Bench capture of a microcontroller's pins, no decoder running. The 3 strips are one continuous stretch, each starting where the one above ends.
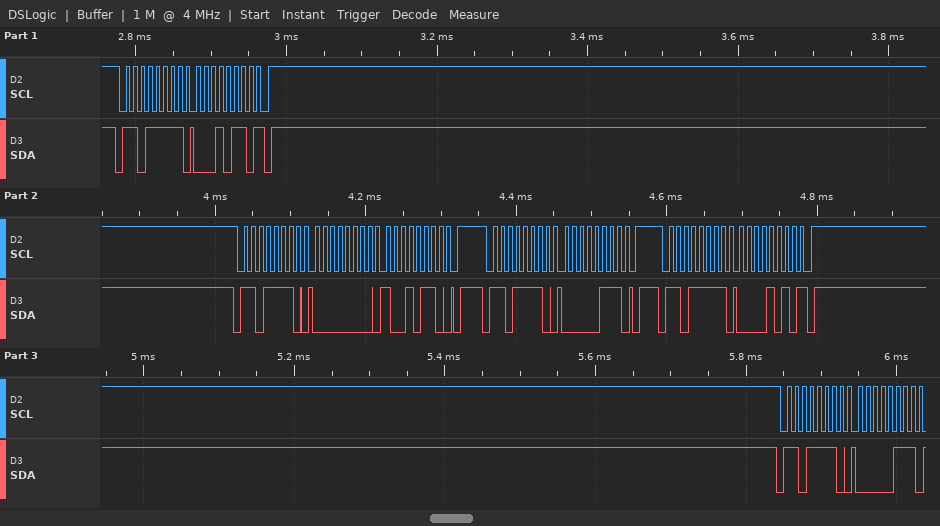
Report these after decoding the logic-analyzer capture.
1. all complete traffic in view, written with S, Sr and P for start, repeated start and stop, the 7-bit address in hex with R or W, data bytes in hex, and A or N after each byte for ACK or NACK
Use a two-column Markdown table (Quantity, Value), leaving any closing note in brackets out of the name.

| Quantity | Value |
|---|---|
| all complete traffic in view, written with S, Sr and P for start, repeated start and stop, the 7-bit address in hex with R or W, data bytes in hex, and A or N after each byte for ACK or NACK | S 6FR A 16 N P S 6FW A 00 A 96 A P S 6FW A 07 A P S 6FR A 0A N P S 6FW A 07 A |
